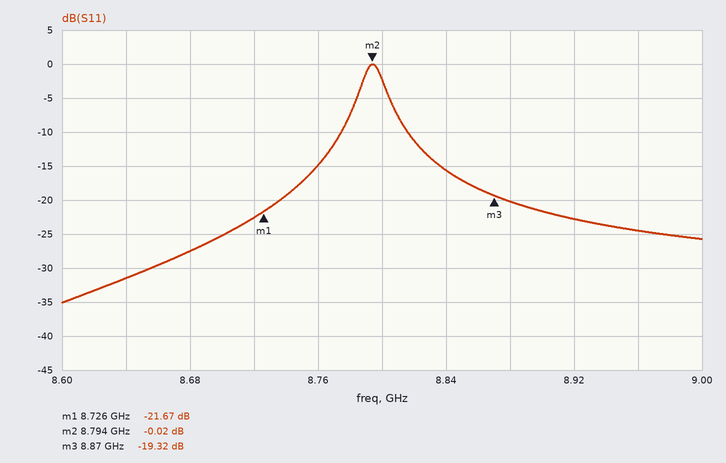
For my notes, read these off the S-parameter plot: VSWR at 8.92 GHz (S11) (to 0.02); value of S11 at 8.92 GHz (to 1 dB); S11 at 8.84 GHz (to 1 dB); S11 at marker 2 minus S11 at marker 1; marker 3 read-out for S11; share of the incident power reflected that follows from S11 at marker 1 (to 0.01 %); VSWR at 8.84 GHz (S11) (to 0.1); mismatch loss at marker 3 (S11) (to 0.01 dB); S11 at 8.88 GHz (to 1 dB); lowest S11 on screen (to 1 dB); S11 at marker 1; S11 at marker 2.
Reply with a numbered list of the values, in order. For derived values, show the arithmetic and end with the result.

1. |Γ| = 10^(-23/20) = 0.0708; VSWR = (1 + 0.0708)/(1 − 0.0708) ≈ 1.15, so 1.16 to the nearest 0.02
2. -23 dB
3. -16 dB
4. -0.02 − (-21.67) = 21.65 dB
5. -19.32 dB
6. 10^(-21.67/10) ≈ 0.68 %
7. |Γ| = 10^(-16/20) = 0.1585; VSWR = (1 + 0.1585)/(1 − 0.1585) ≈ 1.4
8. −10 log10(1 − 10^(-19.32/10)) ≈ 0.05 dB
9. -20 dB
10. -35 dB
11. -21.67 dB
12. -0.02 dB
